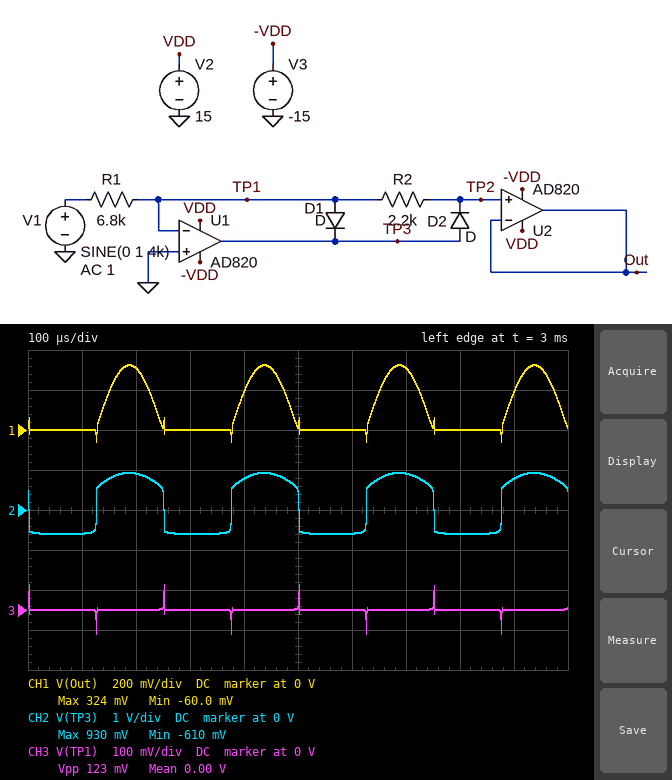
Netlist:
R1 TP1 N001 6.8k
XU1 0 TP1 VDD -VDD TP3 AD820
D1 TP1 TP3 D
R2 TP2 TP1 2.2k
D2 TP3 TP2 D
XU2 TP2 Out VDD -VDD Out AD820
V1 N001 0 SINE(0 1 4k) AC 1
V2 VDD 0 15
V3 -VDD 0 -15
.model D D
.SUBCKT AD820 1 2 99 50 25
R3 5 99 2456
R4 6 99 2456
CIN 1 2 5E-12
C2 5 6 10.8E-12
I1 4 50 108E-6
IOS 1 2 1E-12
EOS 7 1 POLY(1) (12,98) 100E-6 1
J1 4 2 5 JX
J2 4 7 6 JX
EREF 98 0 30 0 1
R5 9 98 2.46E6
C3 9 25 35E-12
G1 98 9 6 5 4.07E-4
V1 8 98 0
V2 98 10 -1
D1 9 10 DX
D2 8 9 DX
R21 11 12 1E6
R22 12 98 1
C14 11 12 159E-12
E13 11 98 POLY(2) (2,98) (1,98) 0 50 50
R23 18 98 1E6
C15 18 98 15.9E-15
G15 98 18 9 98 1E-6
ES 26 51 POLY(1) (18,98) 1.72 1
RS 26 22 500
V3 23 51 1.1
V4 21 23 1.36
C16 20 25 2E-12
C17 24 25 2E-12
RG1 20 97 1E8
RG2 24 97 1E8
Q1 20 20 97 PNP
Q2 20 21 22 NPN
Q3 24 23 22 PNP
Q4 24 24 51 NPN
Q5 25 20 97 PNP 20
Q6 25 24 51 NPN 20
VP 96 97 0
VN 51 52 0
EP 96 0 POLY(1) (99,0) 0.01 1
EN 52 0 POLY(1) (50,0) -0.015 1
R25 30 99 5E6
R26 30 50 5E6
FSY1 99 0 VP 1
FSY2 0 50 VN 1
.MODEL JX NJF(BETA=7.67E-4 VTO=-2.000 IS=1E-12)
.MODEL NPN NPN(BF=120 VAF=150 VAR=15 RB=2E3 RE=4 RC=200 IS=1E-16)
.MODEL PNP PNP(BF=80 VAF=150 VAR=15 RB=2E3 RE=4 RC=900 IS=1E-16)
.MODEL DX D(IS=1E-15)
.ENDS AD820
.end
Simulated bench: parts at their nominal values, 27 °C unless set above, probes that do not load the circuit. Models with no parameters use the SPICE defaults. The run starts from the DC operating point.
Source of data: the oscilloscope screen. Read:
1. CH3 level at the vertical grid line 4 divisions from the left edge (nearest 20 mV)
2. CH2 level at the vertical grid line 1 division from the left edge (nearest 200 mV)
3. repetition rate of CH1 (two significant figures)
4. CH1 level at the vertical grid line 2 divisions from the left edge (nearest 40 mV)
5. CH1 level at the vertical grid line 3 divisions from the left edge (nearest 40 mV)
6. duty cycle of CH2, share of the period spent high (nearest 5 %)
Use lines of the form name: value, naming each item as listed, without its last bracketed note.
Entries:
CH3 level at the vertical grid line 4 divisions from the left edge: 0 V
CH2 level at the vertical grid line 1 division from the left edge: -600 mV
repetition rate of CH1: 4.0 kHz
CH1 level at the vertical grid line 2 divisions from the left edge: 320 mV
CH1 level at the vertical grid line 3 divisions from the left edge: 0 V
duty cycle of CH2, share of the period spent high: 50 %
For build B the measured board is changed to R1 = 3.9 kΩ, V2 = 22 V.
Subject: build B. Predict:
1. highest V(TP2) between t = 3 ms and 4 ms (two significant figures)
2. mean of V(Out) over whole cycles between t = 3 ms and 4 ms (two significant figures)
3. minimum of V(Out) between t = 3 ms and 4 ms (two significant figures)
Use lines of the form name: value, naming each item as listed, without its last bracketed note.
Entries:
highest V(TP2) between t = 3 ms and 4 ms: 560 mV
mean of V(Out) over whole cycles between t = 3 ms and 4 ms: 180 mV
minimum of V(Out) between t = 3 ms and 4 ms: -62 mV
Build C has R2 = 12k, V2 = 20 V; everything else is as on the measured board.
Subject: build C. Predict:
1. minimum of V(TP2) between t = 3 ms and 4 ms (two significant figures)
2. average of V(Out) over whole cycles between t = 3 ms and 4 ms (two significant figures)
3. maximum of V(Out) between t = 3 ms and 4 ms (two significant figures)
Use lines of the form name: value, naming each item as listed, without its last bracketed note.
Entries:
minimum of V(TP2) between t = 3 ms and 4 ms: -61 mV
average of V(Out) over whole cycles between t = 3 ms and 4 ms: 560 mV
maximum of V(Out) between t = 3 ms and 4 ms: 1.8 V
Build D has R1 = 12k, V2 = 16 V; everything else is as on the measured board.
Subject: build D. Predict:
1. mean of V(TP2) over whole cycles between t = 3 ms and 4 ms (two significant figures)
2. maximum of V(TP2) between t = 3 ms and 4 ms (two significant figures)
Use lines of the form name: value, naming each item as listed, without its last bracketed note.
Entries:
mean of V(TP2) over whole cycles between t = 3 ms and 4 ms: 58 mV
maximum of V(TP2) between t = 3 ms and 4 ms: 180 mV
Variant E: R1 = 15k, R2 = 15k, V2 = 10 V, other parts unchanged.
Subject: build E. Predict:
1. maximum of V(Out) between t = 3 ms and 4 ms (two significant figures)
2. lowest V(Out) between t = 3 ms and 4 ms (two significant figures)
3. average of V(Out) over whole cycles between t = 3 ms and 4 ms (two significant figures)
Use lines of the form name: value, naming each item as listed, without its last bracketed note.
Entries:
maximum of V(Out) between t = 3 ms and 4 ms: 1.0 V
lowest V(Out) between t = 3 ms and 4 ms: -59 mV
average of V(Out) over whole cycles between t = 3 ms and 4 ms: 320 mV
